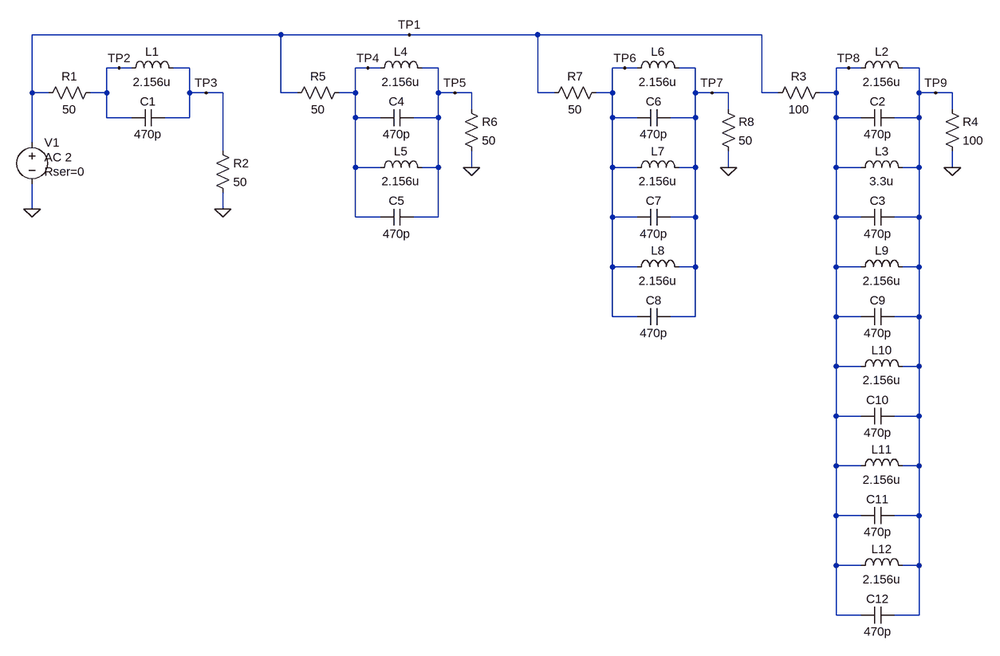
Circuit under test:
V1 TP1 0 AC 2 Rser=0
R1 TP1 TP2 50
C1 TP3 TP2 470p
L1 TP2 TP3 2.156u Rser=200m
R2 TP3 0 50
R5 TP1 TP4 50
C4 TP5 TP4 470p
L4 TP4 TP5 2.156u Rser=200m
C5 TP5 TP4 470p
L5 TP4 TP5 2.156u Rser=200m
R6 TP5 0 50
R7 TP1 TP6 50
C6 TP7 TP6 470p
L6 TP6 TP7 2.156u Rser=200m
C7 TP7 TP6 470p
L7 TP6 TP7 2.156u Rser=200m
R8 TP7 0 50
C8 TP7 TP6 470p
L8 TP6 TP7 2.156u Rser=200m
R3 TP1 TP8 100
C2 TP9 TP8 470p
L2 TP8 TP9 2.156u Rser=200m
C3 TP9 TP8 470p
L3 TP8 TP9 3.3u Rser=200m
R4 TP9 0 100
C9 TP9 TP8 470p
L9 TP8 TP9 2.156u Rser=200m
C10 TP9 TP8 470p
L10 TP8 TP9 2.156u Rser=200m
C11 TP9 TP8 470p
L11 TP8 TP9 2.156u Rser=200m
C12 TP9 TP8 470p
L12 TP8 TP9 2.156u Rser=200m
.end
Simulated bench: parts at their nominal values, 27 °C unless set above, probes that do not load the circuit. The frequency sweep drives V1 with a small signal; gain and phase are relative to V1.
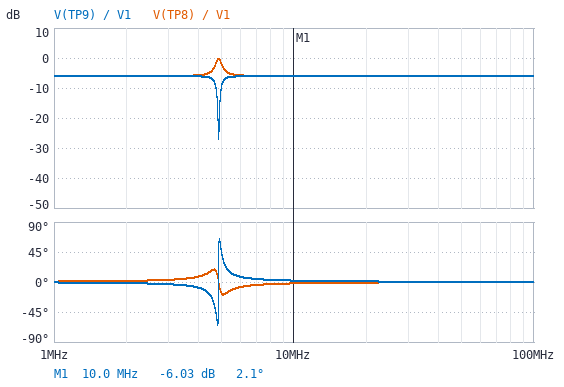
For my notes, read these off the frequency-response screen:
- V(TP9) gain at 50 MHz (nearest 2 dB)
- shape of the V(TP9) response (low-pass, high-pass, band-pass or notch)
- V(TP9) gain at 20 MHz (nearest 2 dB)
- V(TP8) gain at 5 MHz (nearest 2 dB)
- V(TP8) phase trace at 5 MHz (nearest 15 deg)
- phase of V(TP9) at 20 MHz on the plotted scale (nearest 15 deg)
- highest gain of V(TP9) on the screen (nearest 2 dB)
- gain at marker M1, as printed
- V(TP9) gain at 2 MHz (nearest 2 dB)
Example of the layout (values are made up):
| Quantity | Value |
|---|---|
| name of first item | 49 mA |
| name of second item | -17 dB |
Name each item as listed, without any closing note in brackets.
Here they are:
| Quantity | Value |
|---|---|
| V(TP9) gain at 50 MHz | -6 dB |
| shape of the V(TP9) response | notch |
| V(TP9) gain at 20 MHz | -6 dB |
| V(TP8) gain at 5 MHz | -2 dB |
| V(TP8) phase trace at 5 MHz | -15 deg |
| phase of V(TP9) at 20 MHz on the plotted scale | 0 deg |
| highest gain of V(TP9) on the screen | -6 dB |
| gain at marker M1, as printed | -6.03 dB |
| V(TP9) gain at 2 MHz | -6 dB |
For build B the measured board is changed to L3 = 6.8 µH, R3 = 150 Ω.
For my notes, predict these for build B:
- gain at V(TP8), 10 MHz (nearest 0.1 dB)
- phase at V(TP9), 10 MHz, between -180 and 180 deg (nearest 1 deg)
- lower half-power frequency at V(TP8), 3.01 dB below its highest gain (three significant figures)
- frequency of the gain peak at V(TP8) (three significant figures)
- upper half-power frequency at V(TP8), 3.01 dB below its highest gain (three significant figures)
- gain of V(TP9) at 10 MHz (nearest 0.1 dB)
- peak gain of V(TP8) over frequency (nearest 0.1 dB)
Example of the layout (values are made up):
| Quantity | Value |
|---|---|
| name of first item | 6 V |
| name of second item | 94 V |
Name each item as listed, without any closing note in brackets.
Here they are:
| Quantity | Value |
|---|---|
| gain at V(TP8), 10 MHz | -7.9 dB |
| phase at V(TP9), 10 MHz, between -180 and 180 deg | 2 deg |
| lower half-power frequency at V(TP8), 3.01 dB below its highest gain | 4.56 MHz |
| frequency of the gain peak at V(TP8) | 4.71 MHz |
| upper half-power frequency at V(TP8), 3.01 dB below its highest gain | 4.86 MHz |
| gain of V(TP9) at 10 MHz | -8.0 dB |
| peak gain of V(TP8) over frequency | -0.3 dB |
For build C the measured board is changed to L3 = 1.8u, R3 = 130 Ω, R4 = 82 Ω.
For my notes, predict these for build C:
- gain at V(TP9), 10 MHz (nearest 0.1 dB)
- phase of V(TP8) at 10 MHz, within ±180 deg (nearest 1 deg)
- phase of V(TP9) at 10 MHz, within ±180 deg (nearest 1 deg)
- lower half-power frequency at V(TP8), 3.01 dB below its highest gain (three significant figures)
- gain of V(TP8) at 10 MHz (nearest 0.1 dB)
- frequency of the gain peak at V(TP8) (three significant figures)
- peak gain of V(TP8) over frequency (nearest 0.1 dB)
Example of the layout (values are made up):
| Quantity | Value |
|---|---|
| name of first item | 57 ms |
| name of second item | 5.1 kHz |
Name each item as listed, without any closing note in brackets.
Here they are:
| Quantity | Value |
|---|---|
| gain at V(TP9), 10 MHz | -8.3 dB |
| phase of V(TP8) at 10 MHz, within ±180 deg | -3 deg |
| phase of V(TP9) at 10 MHz, within ±180 deg | 2 deg |
| lower half-power frequency at V(TP8), 3.01 dB below its highest gain | 4.91 MHz |
| gain of V(TP8) at 10 MHz | -8.2 dB |
| frequency of the gain peak at V(TP8) | 5.08 MHz |
| peak gain of V(TP8) over frequency | -0.3 dB |
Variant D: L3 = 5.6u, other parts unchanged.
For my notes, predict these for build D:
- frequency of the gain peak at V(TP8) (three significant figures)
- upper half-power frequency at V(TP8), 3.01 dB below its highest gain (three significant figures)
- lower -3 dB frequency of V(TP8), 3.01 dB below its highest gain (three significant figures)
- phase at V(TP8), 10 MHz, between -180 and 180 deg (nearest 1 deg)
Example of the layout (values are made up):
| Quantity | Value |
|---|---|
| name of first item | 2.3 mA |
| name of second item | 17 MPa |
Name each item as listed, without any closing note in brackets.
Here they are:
| Quantity | Value |
|---|---|
| frequency of the gain peak at V(TP8) | 4.74 MHz |
| upper half-power frequency at V(TP8), 3.01 dB below its highest gain | 4.96 MHz |
| lower -3 dB frequency of V(TP8), 3.01 dB below its highest gain | 4.53 MHz |
| phase at V(TP8), 10 MHz, between -180 and 180 deg | -2 deg |
